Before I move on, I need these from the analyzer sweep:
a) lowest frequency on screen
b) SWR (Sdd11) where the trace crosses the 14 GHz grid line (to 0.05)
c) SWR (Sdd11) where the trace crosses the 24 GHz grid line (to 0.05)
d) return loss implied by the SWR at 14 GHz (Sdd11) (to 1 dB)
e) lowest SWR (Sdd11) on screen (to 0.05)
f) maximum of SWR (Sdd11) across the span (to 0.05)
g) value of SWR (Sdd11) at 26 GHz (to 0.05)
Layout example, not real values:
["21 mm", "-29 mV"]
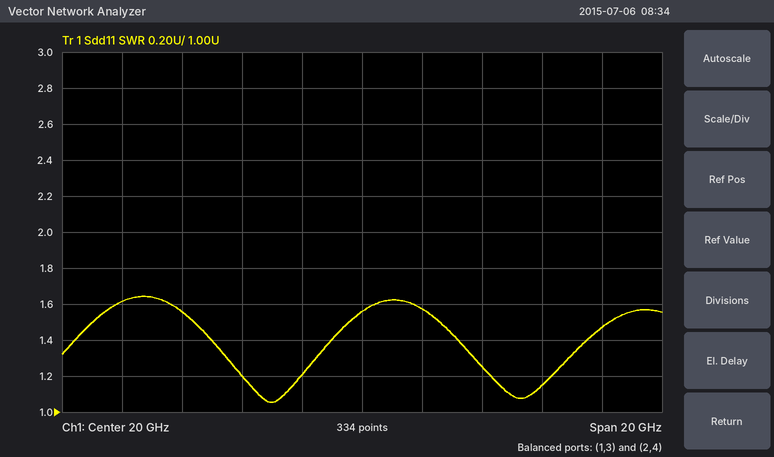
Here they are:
["10 GHz", "1.55", "1.25", "13 dB", "1.05", "1.65", "1.15"]
